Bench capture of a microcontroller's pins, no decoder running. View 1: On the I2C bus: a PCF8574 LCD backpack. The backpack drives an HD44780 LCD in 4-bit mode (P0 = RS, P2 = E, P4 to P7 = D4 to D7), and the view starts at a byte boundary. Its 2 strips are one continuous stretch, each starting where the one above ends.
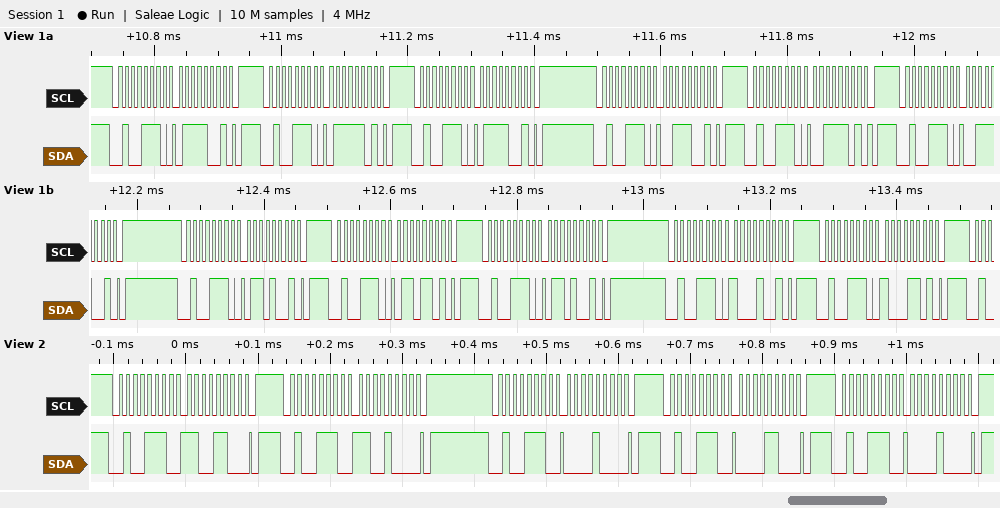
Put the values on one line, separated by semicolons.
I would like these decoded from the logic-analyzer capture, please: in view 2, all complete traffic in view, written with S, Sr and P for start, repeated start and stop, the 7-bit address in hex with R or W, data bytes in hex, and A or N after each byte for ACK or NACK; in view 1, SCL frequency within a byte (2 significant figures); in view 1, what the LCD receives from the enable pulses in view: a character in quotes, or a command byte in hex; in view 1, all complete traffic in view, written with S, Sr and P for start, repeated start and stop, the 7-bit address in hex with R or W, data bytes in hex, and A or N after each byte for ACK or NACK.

S 27W A CC A P S 27W A C8 A P S 27W A 08 A P S 27W A 0C A P S 27W A 08 A P; 100 kHz; 's'; S 27W A 79 A P S 27W A 7D A P S 27W A 79 A P S 27W A 39 A P S 27W A 3D A P S 27W A 39 A P S 27W A 69 A P S 27W A 6D A P S 27W A 69 A P S 27W A 89 A P S 27W A 8D A P
